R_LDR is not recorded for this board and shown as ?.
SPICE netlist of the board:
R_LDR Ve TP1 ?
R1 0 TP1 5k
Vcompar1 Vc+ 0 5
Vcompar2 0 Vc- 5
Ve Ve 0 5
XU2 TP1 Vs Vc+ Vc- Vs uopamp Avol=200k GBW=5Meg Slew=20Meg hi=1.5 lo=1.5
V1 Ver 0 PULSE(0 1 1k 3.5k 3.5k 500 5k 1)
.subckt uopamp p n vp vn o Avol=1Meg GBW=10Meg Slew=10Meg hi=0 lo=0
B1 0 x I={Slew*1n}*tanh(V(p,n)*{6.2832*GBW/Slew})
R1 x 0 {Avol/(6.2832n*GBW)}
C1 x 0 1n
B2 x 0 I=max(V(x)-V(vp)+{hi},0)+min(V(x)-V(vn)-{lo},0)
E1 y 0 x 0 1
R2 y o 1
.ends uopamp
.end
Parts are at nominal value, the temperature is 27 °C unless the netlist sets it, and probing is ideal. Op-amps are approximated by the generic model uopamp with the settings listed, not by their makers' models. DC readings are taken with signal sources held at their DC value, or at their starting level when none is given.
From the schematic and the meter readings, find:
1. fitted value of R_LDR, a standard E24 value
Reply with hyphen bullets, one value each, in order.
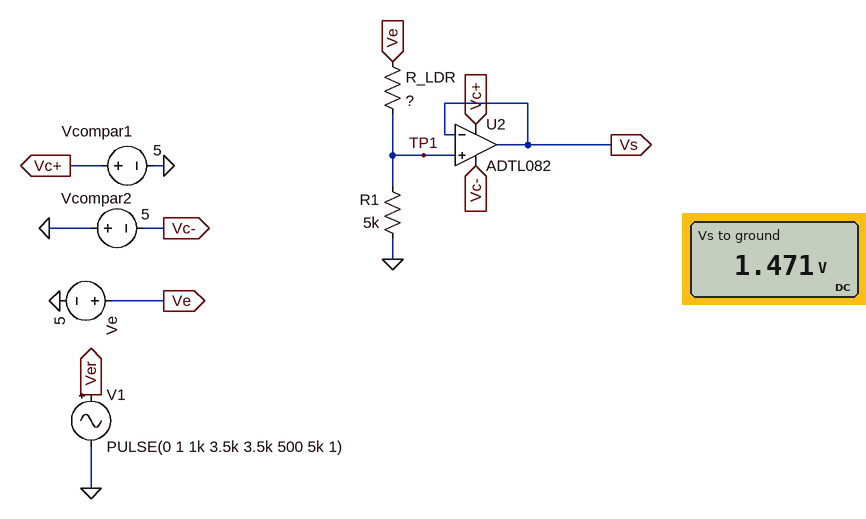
- 12 kΩ
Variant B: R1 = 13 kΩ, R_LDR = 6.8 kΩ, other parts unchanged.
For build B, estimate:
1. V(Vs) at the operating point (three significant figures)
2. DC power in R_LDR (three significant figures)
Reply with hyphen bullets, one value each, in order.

- 3.28 V
- 434 µW
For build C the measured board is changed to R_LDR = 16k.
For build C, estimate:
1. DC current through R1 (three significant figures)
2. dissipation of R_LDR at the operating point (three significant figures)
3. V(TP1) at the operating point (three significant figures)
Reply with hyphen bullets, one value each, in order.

- 238 µA
- 907 µW
- 1.19 V
